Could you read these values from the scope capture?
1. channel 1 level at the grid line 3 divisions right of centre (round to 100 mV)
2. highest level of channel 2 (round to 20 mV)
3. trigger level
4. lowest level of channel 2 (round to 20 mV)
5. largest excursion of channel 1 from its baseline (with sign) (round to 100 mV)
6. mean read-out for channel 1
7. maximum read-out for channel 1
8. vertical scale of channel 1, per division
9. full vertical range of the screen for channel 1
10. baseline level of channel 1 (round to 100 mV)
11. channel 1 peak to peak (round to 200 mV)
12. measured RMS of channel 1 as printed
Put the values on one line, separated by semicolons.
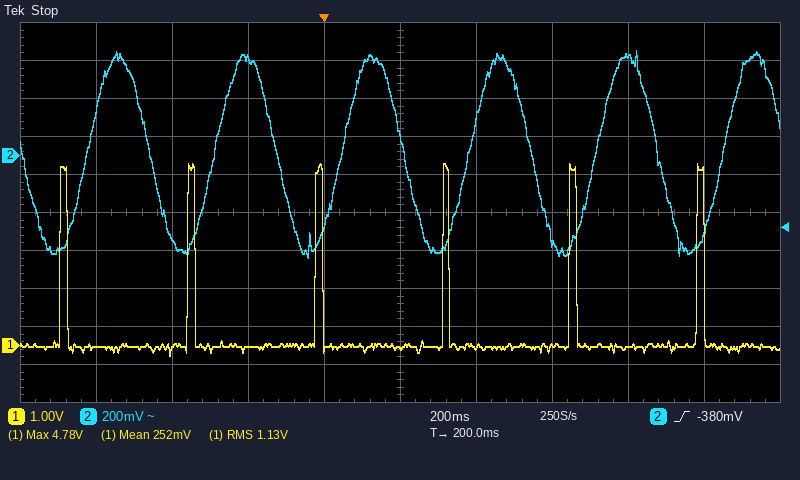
-100 mV; 560 mV; -380 mV; -540 mV; +4.8 V; 252 mV; 4.78 V; 1 V; 10 V; 0.0 V; 5.0 V; 1.13 V
